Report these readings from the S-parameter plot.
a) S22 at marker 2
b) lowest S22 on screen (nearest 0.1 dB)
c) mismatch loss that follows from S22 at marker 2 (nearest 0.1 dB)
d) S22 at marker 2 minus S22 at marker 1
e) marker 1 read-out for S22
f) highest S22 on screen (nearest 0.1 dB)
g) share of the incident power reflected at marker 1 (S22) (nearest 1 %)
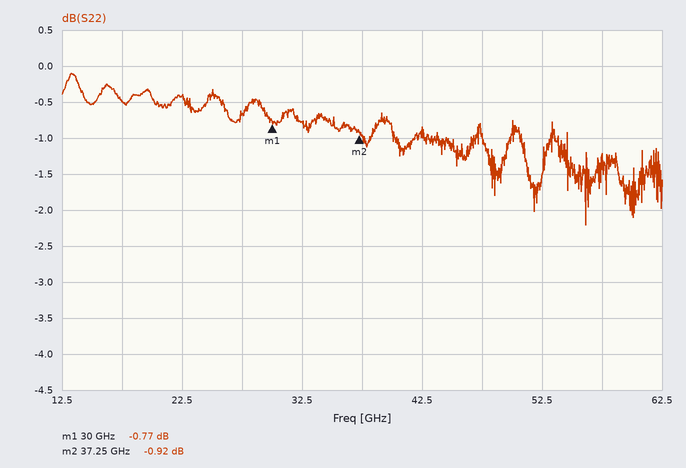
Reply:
-0.92 dB
-2.2 dB
7.2 dB
-0.15 dB
-0.77 dB
-0.1 dB
84 %
